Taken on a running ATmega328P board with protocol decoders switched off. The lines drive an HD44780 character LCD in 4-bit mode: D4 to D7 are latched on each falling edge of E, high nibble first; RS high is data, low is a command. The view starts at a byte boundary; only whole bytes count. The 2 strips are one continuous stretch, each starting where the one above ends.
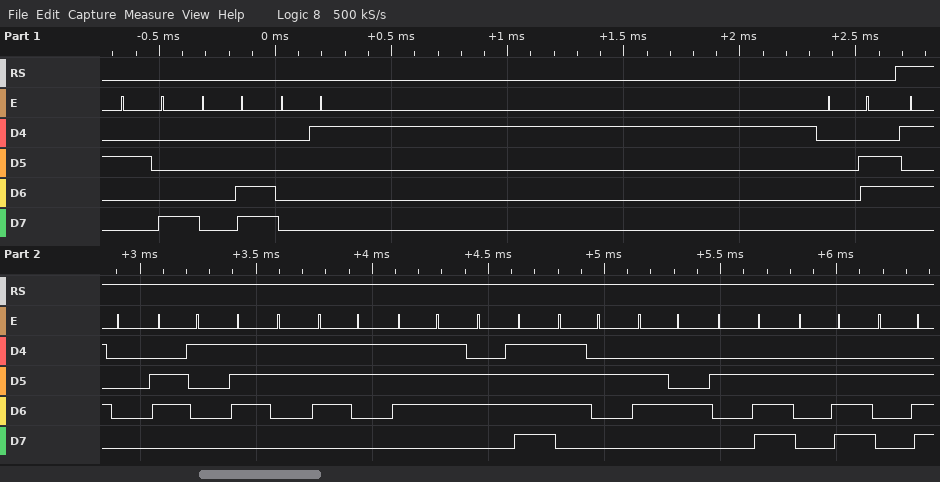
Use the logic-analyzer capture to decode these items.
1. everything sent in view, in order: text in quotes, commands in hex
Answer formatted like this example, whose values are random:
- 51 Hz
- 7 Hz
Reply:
- 0x28 0x0C 0x01 0x06 "Password..."
